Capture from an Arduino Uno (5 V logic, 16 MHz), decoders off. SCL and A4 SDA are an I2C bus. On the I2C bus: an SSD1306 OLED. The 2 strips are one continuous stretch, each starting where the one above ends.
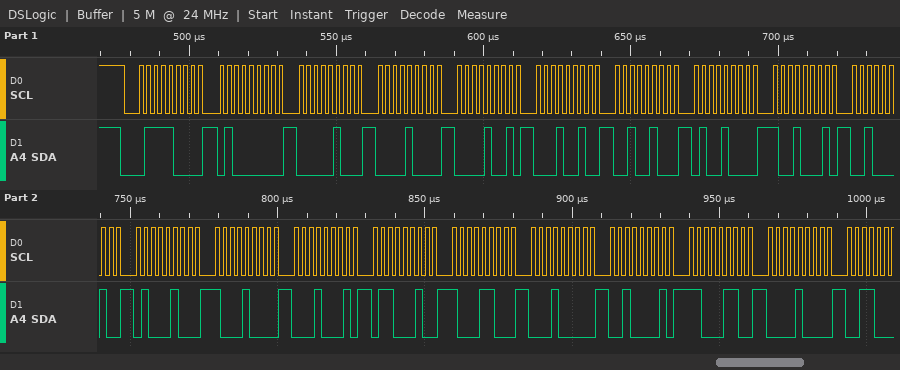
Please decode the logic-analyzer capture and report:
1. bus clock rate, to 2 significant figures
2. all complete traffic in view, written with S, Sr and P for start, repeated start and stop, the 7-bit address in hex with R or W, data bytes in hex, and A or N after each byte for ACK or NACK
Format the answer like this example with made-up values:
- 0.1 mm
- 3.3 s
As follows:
- 400 kHz
- S 3CW A 40 A 04 A 08 A 09 A 12 A 24 A 48 A 91 A 22 A 44 A 88 A 11 A 62 A 8C A 10 A 21 A C6 A 08 A
